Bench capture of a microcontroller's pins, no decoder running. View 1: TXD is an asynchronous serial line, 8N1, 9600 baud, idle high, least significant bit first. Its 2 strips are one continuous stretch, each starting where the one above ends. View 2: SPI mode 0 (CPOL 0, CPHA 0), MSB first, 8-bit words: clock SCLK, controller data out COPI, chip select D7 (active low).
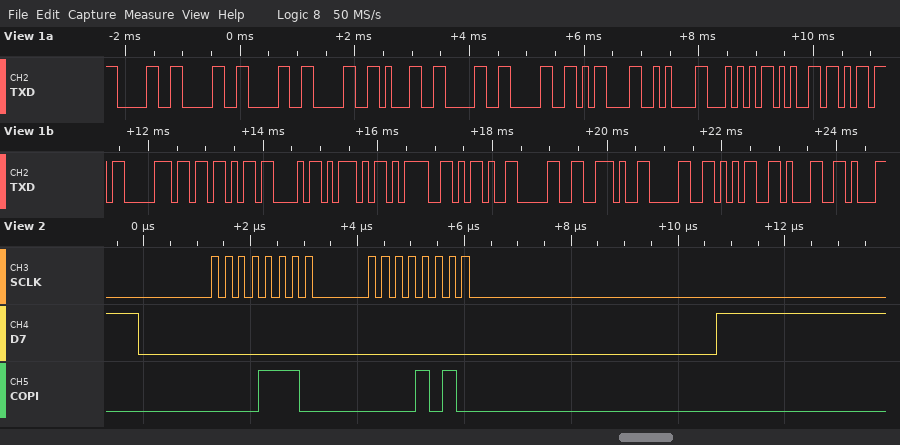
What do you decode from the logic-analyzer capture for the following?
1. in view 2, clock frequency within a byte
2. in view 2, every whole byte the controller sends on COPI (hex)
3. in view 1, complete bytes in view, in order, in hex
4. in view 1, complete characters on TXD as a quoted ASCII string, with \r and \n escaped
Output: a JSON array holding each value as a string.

["4 MHz", "0E 0A", "30 30 30 30 31 30 30 0D 0A 54 65 6D 70 5B 43 5D 3D 2D 30 2E 30 35 31", "\"0000100\\r\\nTemp[C]=-0.051\""]
